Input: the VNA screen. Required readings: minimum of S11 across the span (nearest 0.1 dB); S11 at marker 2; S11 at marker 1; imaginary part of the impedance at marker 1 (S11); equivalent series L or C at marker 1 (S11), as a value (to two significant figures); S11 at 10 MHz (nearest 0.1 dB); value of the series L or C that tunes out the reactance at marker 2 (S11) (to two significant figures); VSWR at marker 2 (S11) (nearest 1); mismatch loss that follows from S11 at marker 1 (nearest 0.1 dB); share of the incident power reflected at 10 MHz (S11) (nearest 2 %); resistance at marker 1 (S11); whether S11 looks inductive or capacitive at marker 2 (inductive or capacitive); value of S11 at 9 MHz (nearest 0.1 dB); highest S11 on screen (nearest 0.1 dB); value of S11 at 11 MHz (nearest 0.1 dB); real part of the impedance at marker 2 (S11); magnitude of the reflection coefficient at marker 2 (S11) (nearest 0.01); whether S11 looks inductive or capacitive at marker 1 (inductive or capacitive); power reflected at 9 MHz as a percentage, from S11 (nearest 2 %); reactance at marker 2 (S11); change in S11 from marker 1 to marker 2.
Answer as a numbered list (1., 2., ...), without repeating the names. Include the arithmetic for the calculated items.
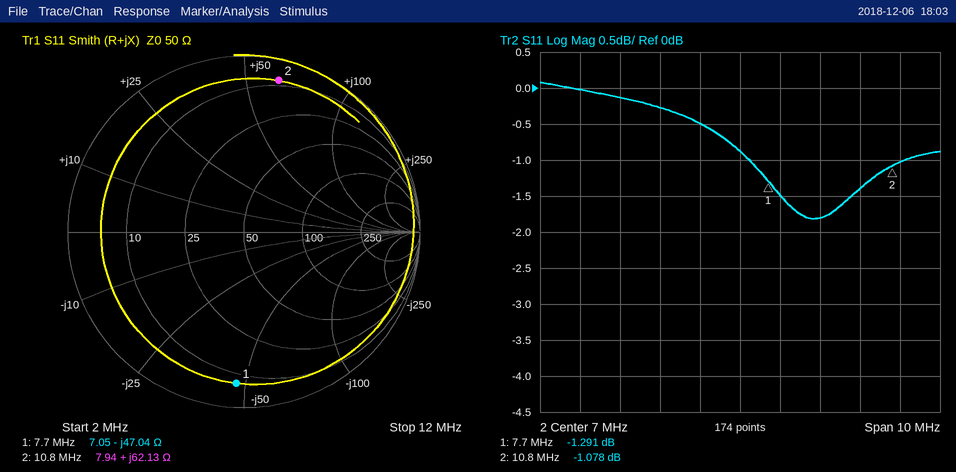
1. -1.8 dB
2. -1.078 dB
3. -1.291 dB
4. -47.04 Ω
5. C = 1/(2π × 7.7 MHz × 47.04 Ω) ≈ 439 pF, so 440 pF to two significant figures
6. -1.4 dB
7. C = 1/(2π × 10.8 MHz × 62.13 Ω) ≈ 237 pF, so 240 pF to two significant figures
8. (1 + 0.8833)/(1 − 0.8833) ≈ 16
9. −10 log10(1 − 10^(-1.291/10)) ≈ 5.9 dB
10. 10^(-1.4/10) ≈ 72 %
11. 7.05 Ω
12. inductive
13. -1.8 dB
14. 0.1 dB
15. -1.0 dB
16. 7.94 Ω
17. 0.88
18. capacitive
19. 10^(-1.8/10) ≈ 66 %
20. +62.13 Ω
21. -1.078 − (-1.291) = 0.213 dB
